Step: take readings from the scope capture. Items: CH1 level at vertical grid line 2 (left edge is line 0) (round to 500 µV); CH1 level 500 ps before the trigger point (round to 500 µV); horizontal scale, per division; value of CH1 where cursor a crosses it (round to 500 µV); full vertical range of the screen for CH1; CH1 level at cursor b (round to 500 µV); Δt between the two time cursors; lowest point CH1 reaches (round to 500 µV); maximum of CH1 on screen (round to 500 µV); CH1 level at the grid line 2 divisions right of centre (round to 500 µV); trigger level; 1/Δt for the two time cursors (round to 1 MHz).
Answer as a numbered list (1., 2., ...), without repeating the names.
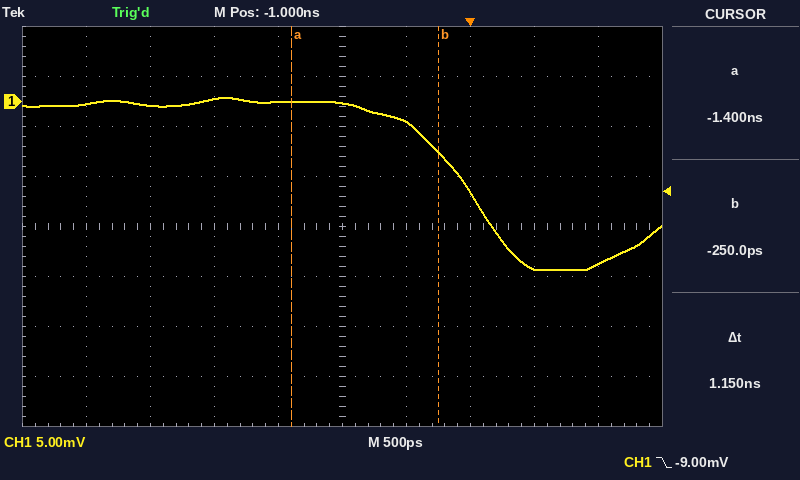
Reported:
1. -500 µV
2. -2.0 mV
3. 500 ps
4. 0.0 mV
5. 40 mV
6. -5.0 mV
7. 1.15 ns
8. -17.0 mV
9. 500 µV
10. -9.0 mV
11. -9.00 mV
12. 870 MHz
